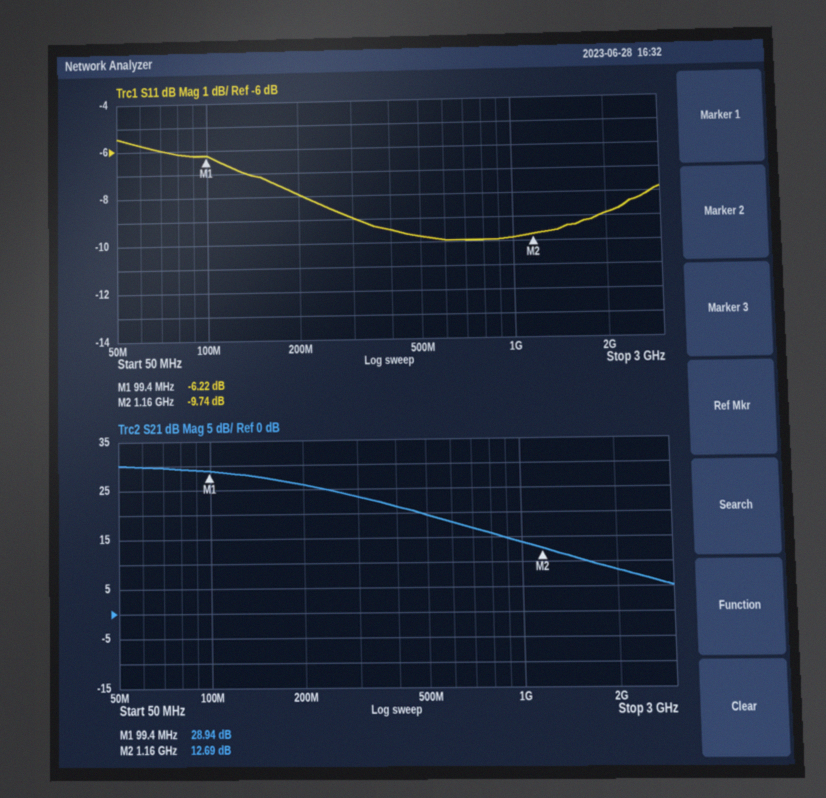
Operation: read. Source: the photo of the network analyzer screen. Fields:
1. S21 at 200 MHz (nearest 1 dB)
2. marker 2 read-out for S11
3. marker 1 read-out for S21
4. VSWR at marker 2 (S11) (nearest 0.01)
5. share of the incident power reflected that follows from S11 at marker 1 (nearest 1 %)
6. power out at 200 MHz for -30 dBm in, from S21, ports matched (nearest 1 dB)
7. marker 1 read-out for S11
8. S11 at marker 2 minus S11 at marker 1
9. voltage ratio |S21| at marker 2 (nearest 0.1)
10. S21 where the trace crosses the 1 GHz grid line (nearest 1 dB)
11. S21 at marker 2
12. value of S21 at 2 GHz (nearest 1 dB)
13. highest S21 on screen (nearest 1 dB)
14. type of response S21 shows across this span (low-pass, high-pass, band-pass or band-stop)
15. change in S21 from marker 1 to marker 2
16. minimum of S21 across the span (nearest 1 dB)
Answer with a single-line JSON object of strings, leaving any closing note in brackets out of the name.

{"S21 at 200 MHz": "26 dB", "marker 2 read-out for S11": "-9.74 dB", "marker 1 read-out for S21": "28.94 dB", "VSWR at marker 2 (S11)": "1.97", "share of the incident power reflected that follows from S11 at marker 1": "24 %", "power out at 200 MHz for -30 dBm in, from S21, ports matched": "-4 dBm", "marker 1 read-out for S11": "-6.22 dB", "S11 at marker 2 minus S11 at marker 1": "-3.52 dB", "voltage ratio |S21| at marker 2": "4.3", "S21 where the trace crosses the 1 GHz grid line": "14 dB", "S21 at marker 2": "12.69 dB", "value of S21 at 2 GHz": "8 dB", "highest S21 on screen": "30 dB", "type of response S21 shows across this span": "low-pass", "change in S21 from marker 1 to marker 2": "-16.25 dB", "minimum of S21 across the span": "5 dB"}
